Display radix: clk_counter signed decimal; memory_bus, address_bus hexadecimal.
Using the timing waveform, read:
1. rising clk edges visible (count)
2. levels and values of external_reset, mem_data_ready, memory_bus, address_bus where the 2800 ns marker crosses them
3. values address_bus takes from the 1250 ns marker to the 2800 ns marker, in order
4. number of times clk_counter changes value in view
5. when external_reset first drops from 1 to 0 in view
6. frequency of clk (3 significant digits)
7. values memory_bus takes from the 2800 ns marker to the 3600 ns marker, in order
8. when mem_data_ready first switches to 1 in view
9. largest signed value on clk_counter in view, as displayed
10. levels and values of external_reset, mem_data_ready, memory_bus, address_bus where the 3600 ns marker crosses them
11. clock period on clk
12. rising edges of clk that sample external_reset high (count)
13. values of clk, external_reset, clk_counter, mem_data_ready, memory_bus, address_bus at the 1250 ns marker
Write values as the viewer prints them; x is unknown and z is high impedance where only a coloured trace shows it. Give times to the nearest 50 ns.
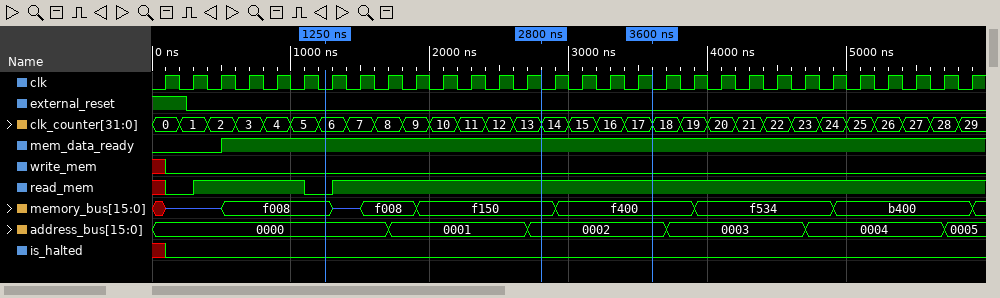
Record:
30
external_reset=0, mem_data_ready=1, memory_bus=f150, address_bus=0002
0000, 0001, 0002
29
250 ns
5.00 MHz
f150, f400
500 ns
29
external_reset=0, mem_data_ready=1, memory_bus=f400, address_bus=0002
200 ns
1
clk=0, external_reset=0, clk_counter=6, mem_data_ready=1, memory_bus=f008, address_bus=0000
